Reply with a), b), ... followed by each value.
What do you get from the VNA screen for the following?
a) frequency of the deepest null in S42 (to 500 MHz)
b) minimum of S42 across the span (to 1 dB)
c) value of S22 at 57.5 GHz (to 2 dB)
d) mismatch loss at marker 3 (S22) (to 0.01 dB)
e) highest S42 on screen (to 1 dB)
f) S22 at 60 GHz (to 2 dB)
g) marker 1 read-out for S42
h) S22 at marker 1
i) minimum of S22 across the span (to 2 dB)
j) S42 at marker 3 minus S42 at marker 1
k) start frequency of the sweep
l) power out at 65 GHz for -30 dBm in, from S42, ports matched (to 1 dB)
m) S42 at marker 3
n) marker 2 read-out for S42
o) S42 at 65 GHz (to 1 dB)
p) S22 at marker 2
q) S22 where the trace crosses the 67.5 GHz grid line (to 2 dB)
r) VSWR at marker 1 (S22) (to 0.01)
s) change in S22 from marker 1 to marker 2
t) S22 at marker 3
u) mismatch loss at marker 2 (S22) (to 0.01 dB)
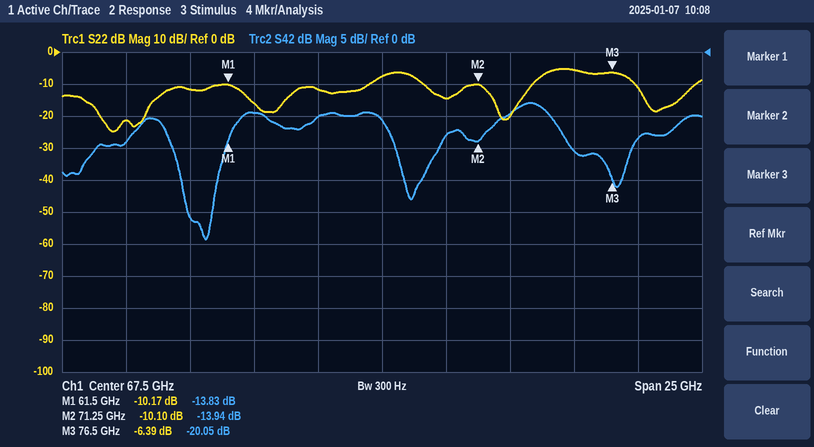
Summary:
a) 60.5 GHz
b) -29 dB
c) -22 dB
d) 1.13 dB
e) -8 dB
f) -12 dB
g) -13.83 dB
h) -10.17 dB
i) -24 dB
j) -6.22 dB
k) 55 GHz
l) -40 dBm
m) -20.05 dB
n) -13.94 dB
o) -10 dB
p) -10.10 dB
q) -8 dB
r) 1.90
s) 0.07 dB
t) -6.39 dB
u) 0.45 dB
